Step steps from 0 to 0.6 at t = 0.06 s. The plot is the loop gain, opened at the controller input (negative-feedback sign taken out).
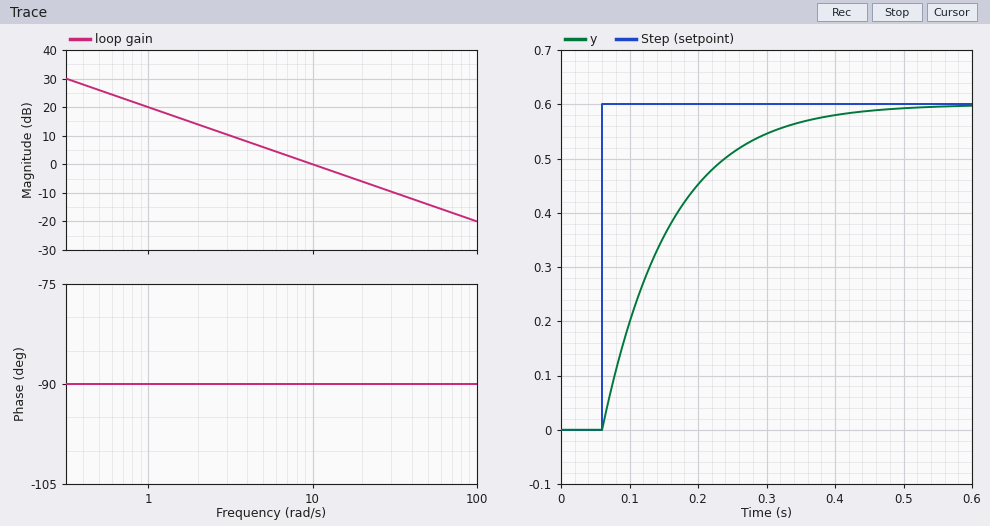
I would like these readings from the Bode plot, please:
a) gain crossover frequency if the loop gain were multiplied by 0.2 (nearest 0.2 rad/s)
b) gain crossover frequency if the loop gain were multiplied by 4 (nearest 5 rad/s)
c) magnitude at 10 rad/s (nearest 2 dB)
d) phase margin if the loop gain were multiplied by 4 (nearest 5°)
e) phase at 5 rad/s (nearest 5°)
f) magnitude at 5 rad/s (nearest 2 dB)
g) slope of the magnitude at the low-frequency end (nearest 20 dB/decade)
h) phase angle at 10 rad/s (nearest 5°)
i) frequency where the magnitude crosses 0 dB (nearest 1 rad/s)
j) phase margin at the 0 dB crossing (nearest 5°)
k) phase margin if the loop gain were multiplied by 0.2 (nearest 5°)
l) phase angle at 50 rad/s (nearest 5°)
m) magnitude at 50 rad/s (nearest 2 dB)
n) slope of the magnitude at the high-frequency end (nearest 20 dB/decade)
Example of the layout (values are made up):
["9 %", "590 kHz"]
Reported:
["2.0 rad/s", "40 rad/s", "0 dB", "90°", "-90°", "6 dB", "-20 dB/decade", "-90°", "10 rad/s", "90°", "90°", "-90°", "-14 dB", "-20 dB/decade"]
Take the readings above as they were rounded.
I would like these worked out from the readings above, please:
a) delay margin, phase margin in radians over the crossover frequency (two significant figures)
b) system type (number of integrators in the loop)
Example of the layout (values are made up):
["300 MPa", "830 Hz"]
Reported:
["0.16 s", "1"]
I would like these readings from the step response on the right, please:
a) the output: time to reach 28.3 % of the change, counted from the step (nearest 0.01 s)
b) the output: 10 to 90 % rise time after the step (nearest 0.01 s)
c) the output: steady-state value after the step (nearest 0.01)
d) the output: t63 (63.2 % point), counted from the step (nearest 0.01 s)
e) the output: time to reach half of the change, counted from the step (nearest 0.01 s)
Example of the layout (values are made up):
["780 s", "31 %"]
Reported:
["0.03 s", "0.22 s", "0.60", "0.10 s", "0.07 s"]
